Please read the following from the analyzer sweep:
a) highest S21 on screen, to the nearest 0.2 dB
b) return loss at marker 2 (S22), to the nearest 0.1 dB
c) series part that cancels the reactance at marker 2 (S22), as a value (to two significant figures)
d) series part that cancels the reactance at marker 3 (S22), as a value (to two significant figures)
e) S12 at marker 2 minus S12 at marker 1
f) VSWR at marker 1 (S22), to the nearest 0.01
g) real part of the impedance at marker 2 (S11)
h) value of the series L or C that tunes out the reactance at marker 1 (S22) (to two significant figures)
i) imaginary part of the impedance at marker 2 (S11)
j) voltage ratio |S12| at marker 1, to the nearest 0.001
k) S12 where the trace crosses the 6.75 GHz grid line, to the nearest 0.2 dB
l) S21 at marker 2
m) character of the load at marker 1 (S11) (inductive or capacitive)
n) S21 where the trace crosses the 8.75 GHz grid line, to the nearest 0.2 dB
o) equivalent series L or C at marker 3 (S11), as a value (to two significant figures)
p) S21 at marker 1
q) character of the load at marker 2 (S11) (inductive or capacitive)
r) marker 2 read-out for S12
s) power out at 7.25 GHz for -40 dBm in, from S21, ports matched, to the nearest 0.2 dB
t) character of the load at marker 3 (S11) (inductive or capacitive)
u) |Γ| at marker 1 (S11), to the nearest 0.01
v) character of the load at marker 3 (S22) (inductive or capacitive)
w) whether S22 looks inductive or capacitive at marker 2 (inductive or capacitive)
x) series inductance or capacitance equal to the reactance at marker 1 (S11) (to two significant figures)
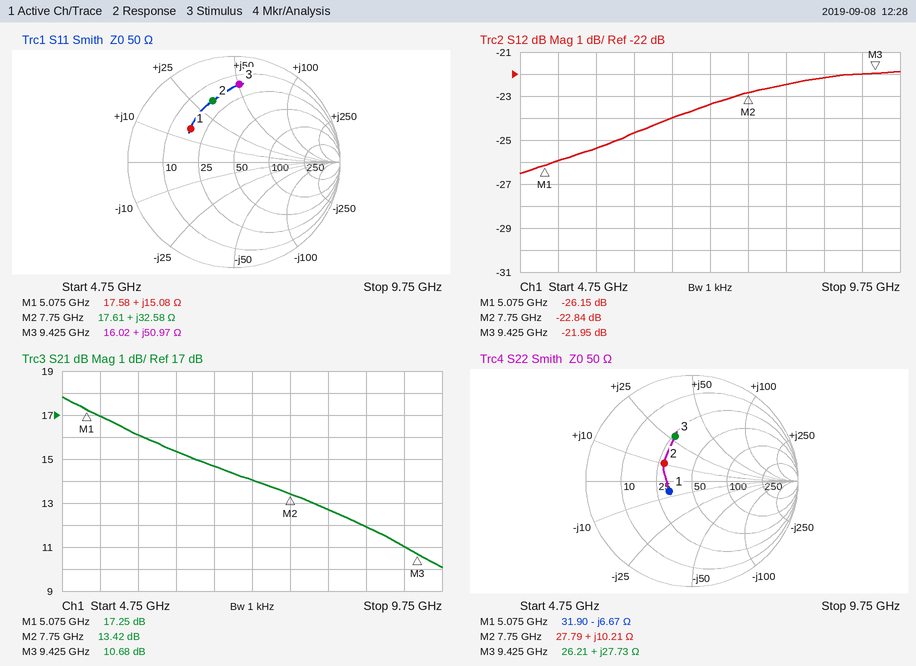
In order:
17.8 dB
10.1 dB
2.0 pF
610 fF
3.31 dB
1.61
17.61 Ω
210 pH
+32.58 Ω
0.049
-24.0 dB
13.42 dB
inductive
12.0 dB
860 pH
17.25 dB
inductive
-22.84 dB
-26.0 dBm
inductive
0.52
inductive
inductive
470 pH
